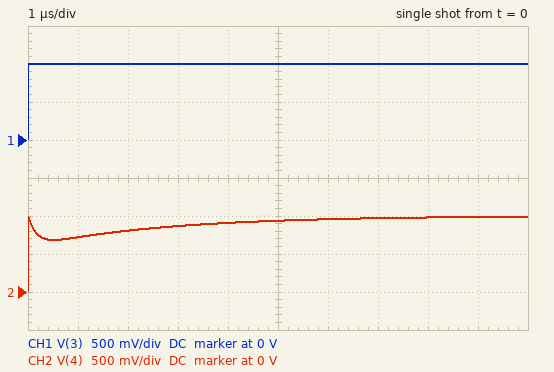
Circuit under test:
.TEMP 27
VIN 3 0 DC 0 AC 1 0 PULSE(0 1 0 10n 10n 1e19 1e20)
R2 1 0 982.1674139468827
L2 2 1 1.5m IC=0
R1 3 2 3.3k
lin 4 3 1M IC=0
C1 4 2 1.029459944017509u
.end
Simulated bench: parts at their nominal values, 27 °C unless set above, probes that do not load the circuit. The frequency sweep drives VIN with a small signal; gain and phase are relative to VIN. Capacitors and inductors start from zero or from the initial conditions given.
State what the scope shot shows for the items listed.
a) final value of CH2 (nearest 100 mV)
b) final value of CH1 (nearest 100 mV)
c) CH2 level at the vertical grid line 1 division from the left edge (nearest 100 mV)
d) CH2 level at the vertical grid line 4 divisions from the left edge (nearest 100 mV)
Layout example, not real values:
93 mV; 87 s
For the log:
1.0 V; 1.0 V; 700 mV; 900 mV
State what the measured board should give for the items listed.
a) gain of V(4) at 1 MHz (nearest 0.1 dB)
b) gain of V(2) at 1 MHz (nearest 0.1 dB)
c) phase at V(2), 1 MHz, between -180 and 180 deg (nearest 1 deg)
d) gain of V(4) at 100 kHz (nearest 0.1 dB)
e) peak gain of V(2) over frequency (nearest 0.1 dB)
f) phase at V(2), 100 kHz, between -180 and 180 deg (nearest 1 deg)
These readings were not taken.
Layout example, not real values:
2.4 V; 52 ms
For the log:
-1.6 dB; -1.6 dB; 12 deg; -2.9 dB; 0 dB; -11 deg
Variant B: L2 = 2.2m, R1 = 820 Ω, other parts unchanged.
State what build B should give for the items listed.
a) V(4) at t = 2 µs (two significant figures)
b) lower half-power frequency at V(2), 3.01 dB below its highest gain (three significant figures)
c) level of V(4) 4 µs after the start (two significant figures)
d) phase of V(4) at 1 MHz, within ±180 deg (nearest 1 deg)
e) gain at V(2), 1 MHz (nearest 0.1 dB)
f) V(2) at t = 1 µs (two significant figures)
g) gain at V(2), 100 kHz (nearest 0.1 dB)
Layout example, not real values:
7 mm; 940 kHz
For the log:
820 mV; 220 Hz; 890 mV; 3 deg; -0.1 dB; 830 mV; -2.2 dB
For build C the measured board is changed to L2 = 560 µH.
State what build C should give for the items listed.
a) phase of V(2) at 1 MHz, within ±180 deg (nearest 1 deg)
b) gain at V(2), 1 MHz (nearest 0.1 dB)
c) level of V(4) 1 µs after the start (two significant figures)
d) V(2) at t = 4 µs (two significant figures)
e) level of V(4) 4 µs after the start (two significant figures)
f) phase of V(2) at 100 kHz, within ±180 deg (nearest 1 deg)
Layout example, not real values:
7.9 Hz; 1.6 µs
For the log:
21 deg; -4.4 dB; 660 mV; 930 mV; 940 mV; -21 deg
